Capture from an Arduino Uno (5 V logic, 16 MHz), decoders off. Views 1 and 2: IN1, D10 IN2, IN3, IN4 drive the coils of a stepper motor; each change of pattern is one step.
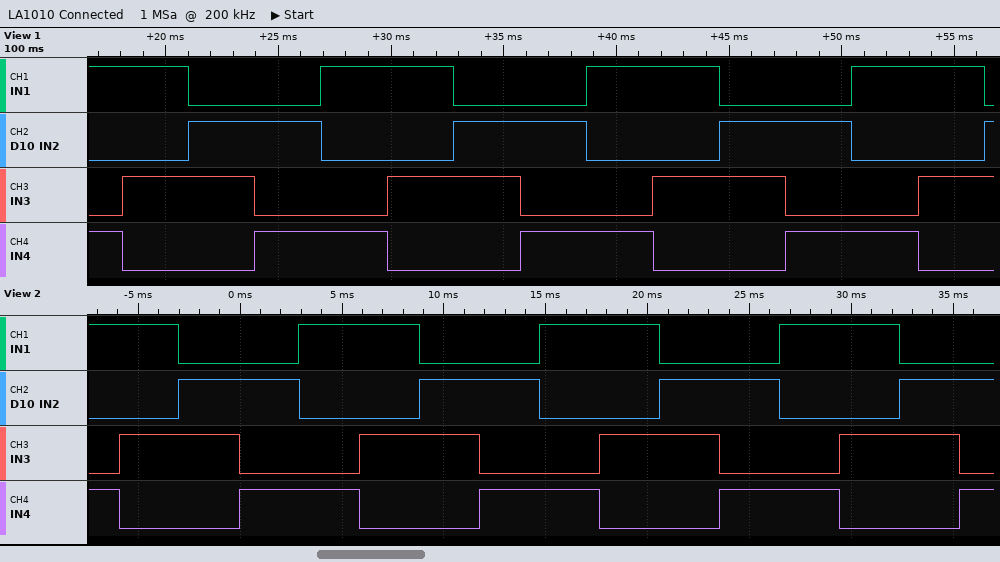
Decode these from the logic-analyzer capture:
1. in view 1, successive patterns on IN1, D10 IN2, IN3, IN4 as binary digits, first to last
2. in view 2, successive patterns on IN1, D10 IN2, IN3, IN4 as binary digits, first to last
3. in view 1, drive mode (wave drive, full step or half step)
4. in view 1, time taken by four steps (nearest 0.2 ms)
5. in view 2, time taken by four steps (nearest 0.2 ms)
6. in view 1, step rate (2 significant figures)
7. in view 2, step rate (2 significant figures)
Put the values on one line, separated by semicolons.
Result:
1001 1010 0110 0101 1001 1010 0110 0101 1001 1010 0110 0101 1001 1010 0110; 1001 1010 0110 0101 1001 1010 0110 0101 1001 1010 0110 0101 1001 1010 0110 0101; full step; 11.8 ms; 11.8 ms; 340 steps/s; 340 steps/s
